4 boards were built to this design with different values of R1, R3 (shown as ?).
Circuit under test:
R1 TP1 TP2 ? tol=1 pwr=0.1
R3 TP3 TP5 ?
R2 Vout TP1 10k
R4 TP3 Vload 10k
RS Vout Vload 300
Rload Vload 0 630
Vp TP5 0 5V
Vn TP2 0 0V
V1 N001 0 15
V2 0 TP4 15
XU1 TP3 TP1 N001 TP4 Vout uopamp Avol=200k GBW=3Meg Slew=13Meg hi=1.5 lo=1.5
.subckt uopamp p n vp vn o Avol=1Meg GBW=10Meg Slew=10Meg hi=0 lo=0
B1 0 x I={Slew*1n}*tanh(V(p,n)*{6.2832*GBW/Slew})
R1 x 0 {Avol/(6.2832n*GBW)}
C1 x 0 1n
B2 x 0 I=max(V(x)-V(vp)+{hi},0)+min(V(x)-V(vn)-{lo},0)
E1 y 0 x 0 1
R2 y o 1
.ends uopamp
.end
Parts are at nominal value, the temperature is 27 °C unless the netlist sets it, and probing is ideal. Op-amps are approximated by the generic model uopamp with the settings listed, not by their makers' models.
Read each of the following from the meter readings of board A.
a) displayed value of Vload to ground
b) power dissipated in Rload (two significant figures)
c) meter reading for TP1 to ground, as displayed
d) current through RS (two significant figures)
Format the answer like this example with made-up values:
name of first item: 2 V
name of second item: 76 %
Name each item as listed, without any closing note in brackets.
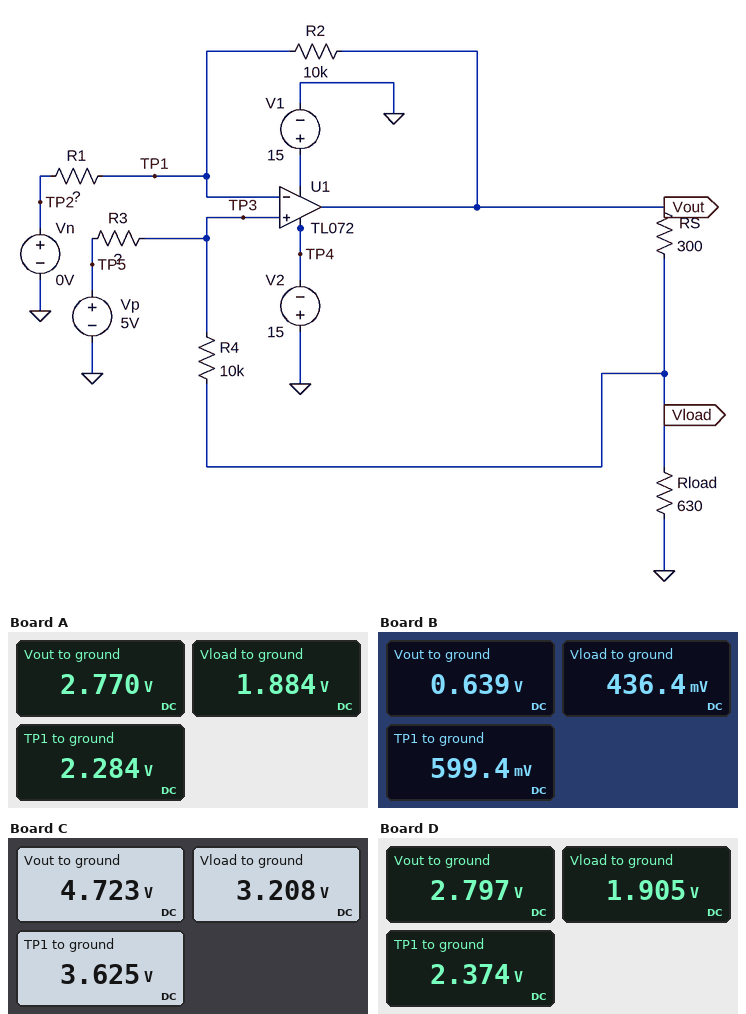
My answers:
displayed value of Vload to ground: 1.884 V
power dissipated in Rload: 5.6 mW
meter reading for TP1 to ground, as displayed: 2.284 V
current through RS: 3.0 mA
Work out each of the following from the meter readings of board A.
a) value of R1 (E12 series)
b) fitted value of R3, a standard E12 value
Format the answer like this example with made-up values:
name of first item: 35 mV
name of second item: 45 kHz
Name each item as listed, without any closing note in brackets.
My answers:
value of R1: 47 kΩ
fitted value of R3, a standard E12 value: 68 kΩ
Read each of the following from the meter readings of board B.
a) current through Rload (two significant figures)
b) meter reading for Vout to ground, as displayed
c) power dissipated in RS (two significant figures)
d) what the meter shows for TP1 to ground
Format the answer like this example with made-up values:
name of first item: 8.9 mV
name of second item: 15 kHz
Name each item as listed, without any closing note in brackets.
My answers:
current through Rload: 690 µA
meter reading for Vout to ground, as displayed: 0.639 V
power dissipated in RS: 140 µW
what the meter shows for TP1 to ground: 599.4 mV
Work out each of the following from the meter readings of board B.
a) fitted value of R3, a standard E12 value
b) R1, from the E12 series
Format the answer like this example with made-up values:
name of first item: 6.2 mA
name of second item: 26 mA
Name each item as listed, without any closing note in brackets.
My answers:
fitted value of R3, a standard E12 value: 270 kΩ
R1, from the E12 series: 150 kΩ
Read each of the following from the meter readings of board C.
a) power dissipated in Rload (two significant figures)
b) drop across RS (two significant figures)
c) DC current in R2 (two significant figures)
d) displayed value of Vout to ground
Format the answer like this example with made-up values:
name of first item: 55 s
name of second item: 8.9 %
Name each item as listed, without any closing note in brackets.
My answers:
power dissipated in Rload: 16 mW
drop across RS: 1.5 V
DC current in R2: 110 µA
displayed value of Vout to ground: 4.723 V
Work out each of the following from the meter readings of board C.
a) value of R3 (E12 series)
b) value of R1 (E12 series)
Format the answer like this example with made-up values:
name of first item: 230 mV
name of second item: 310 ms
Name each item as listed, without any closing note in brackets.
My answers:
value of R3: 33 kΩ
value of R1: 33 kΩ
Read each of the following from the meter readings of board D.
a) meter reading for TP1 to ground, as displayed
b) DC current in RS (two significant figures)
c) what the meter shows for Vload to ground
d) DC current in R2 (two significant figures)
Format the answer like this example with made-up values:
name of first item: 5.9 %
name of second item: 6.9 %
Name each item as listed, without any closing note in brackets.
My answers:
meter reading for TP1 to ground, as displayed: 2.374 V
DC current in RS: 3.0 mA
what the meter shows for Vload to ground: 1.905 V
DC current in R2: 42 µA
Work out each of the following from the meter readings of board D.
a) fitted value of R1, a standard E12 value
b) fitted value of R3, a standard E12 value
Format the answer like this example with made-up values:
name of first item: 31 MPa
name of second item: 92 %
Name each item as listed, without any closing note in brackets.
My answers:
fitted value of R1, a standard E12 value: 56 kΩ
fitted value of R3, a standard E12 value: 56 kΩ
